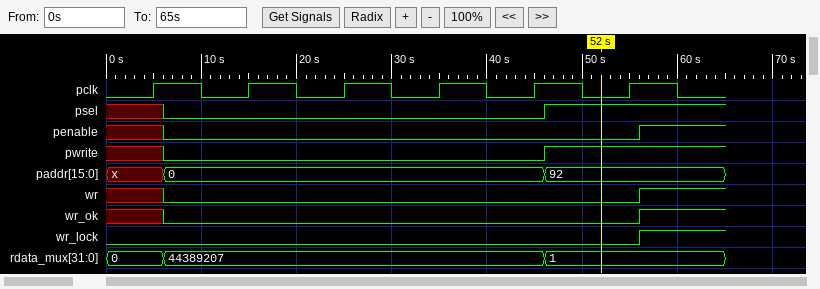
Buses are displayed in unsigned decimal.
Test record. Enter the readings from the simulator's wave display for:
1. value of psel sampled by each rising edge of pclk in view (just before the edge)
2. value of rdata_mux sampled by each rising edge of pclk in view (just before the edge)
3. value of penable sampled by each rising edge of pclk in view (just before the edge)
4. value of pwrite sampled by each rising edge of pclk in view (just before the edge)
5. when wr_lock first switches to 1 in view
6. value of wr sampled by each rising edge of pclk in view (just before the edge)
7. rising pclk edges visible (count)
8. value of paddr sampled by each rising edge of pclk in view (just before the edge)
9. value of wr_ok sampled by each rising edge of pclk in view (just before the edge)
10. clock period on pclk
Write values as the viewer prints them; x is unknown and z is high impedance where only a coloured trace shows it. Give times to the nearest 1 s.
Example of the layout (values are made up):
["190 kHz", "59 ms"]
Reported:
["x 0 0 0 0 1", "0, 44389207, 44389207, 44389207, 44389207, 1", "x 0 0 0 0 0", "x 0 0 0 0 1", "56 s", "x 0 0 0 0 0", "6", "x, 0, 0, 0, 0, 92", "x 0 0 0 0 0", "10 s"]
